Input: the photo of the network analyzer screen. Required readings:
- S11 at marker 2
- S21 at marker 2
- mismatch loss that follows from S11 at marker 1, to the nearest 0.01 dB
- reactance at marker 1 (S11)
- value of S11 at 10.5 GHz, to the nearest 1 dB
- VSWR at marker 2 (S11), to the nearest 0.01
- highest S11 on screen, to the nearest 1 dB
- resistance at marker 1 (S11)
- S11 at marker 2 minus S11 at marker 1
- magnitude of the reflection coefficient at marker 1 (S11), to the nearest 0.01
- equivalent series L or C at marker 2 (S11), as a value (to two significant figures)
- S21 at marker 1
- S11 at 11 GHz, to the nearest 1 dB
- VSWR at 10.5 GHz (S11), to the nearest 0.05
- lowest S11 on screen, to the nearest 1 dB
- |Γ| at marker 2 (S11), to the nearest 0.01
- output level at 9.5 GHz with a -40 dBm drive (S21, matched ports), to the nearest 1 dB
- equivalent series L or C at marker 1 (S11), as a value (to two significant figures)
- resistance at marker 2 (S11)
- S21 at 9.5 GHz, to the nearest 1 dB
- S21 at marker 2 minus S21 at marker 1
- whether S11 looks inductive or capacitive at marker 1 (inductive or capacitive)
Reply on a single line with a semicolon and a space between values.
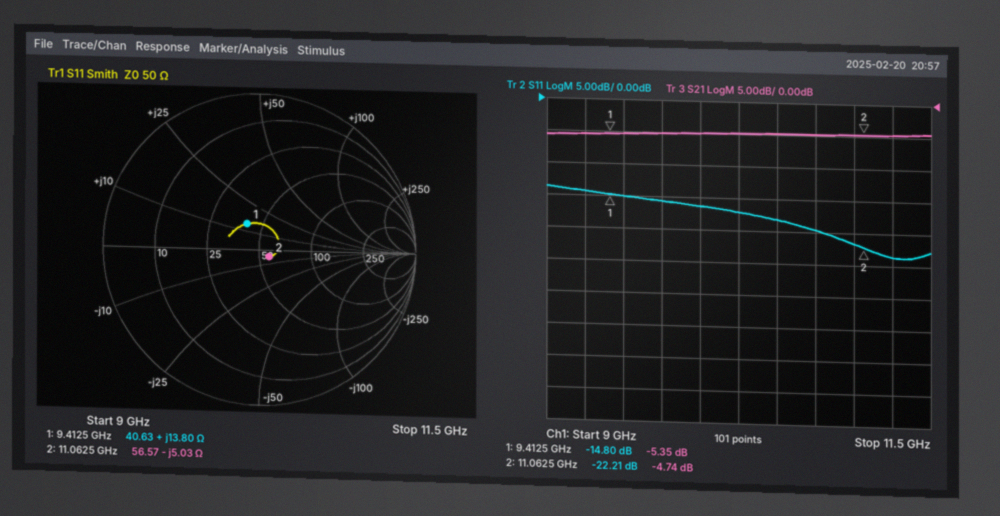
-22.21 dB; -4.74 dB; 0.15 dB; +13.80 Ω; -18 dB; 1.17; -14 dB; 40.63 Ω; -7.41 dB; 0.18; 2.9 pF; -5.35 dB; -22 dB; 1.30; -24 dB; 0.08; -45 dBm; 230 pH; 56.57 Ω; -5 dB; 0.61 dB; inductive
